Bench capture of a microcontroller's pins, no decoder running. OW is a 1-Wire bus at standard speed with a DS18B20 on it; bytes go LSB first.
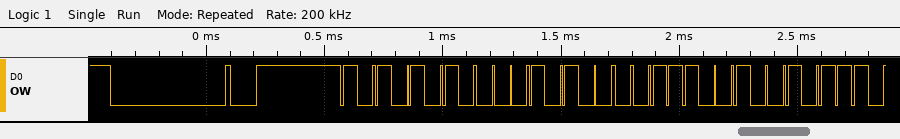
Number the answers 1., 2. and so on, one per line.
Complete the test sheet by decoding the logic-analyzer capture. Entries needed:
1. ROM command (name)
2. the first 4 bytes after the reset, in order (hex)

1. Match ROM
2. 55 28 9C 74
